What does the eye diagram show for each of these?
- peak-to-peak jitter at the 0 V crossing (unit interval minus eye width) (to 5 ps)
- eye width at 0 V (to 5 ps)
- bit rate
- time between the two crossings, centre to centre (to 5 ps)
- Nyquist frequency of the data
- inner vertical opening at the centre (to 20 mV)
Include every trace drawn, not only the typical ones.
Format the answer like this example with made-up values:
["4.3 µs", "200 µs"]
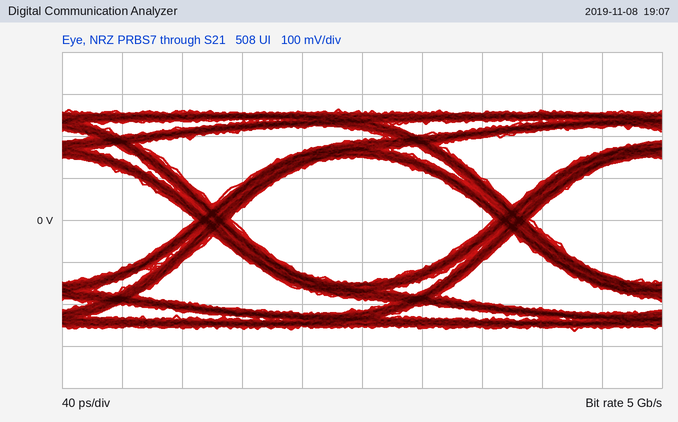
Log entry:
["25 ps", "175 ps", "5 Gb/s", "200 ps", "2.5 GHz", "300 mV"]
